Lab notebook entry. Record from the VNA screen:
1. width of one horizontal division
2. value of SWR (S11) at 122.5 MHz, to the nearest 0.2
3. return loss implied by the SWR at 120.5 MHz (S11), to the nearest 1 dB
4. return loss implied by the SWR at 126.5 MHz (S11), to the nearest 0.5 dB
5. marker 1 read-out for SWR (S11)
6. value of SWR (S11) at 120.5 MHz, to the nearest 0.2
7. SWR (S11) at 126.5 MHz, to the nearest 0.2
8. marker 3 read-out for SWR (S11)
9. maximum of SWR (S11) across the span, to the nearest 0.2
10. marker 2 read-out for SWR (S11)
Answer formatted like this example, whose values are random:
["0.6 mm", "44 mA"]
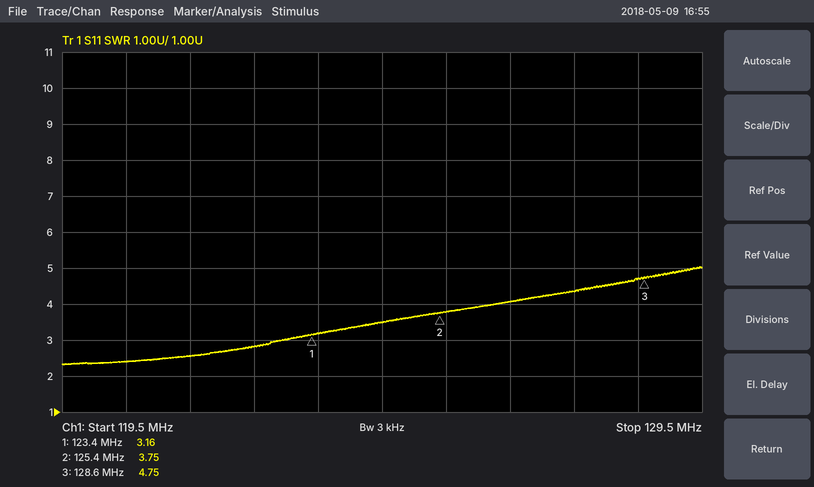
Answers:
["1 MHz", "2.8", "8 dB", "4.5 dB", "3.16", "2.4", "4.0", "4.75", "5.0", "3.75"]
